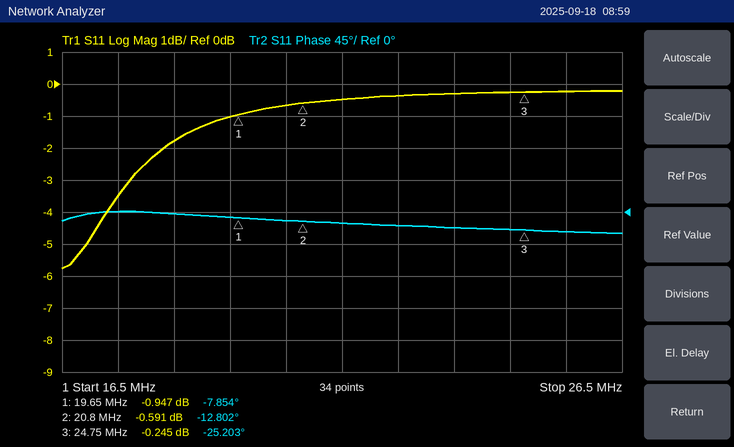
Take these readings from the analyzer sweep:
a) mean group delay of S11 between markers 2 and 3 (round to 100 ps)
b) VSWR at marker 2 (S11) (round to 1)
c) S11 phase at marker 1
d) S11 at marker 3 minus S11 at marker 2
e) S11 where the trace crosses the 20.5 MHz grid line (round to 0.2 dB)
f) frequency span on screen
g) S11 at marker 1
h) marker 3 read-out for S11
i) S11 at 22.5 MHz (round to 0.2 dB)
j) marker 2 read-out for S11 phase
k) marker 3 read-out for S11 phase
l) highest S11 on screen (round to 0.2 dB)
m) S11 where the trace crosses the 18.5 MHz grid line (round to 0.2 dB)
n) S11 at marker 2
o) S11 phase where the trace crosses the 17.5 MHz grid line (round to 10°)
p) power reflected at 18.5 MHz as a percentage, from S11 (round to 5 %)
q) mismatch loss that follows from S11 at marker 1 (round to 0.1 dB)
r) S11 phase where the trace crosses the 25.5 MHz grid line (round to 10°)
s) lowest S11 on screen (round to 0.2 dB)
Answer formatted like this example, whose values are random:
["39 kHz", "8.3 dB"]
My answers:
["8.7 ns", "29", "-7.854°", "0.346 dB", "-0.6 dB", "10 MHz", "-0.947 dB", "-0.245 dB", "-0.4 dB", "-12.802°", "-25.203°", "-0.2 dB", "-1.8 dB", "-0.591 dB", "0°", "65 %", "7.1 dB", "-30°", "-5.8 dB"]
